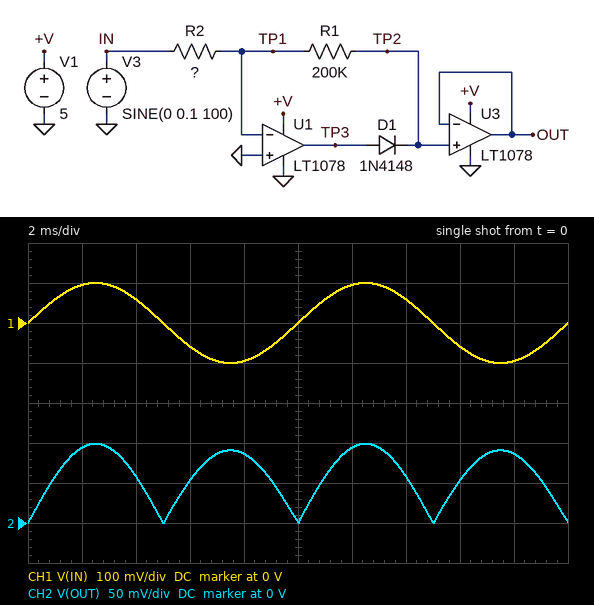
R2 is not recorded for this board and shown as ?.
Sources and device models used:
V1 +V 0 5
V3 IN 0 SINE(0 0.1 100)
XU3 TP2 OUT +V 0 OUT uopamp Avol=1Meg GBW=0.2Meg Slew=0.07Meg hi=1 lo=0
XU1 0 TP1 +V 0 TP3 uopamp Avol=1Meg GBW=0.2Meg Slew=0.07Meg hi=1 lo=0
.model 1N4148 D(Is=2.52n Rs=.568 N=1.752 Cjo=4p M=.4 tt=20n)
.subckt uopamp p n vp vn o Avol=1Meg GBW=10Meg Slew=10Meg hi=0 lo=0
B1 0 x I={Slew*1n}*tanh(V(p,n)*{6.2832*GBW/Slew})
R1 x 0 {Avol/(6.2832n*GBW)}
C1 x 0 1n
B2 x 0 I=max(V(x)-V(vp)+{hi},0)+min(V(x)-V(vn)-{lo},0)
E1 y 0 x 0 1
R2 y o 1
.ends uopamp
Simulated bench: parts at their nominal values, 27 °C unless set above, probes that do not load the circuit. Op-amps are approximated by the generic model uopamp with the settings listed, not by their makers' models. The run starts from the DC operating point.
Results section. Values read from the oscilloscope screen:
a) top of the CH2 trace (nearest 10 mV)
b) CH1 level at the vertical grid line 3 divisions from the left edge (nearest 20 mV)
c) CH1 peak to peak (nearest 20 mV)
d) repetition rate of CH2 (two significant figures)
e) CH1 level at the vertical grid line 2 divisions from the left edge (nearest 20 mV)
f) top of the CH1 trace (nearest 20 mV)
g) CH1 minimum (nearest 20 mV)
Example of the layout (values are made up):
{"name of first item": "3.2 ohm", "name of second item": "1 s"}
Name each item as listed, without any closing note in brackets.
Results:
{"top of the CH2 trace": "100 mV", "CH1 level at the vertical grid line 3 divisions from the left edge": "-60 mV", "CH1 peak to peak": "200 mV", "repetition rate of CH2": "200 Hz", "CH1 level at the vertical grid line 2 divisions from the left edge": "60 mV", "top of the CH1 trace": "100 mV", "CH1 minimum": "-100 mV"}
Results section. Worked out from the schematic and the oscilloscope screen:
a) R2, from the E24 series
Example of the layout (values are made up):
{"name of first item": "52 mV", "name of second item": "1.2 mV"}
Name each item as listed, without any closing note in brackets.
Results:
{"R2, from the E24 series": "220 kΩ"}
